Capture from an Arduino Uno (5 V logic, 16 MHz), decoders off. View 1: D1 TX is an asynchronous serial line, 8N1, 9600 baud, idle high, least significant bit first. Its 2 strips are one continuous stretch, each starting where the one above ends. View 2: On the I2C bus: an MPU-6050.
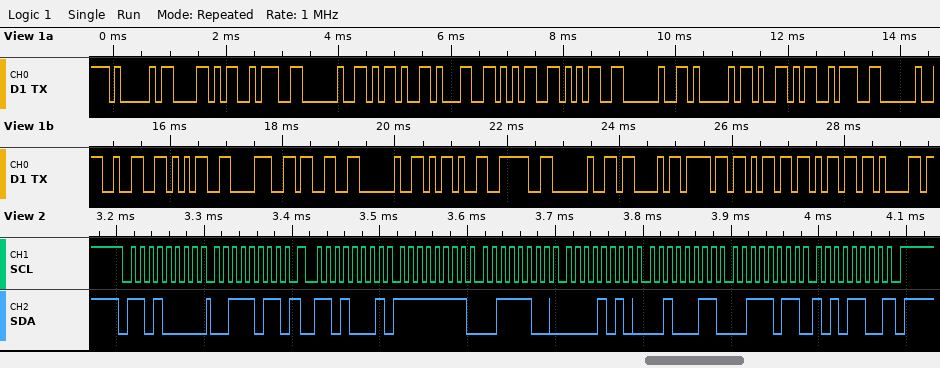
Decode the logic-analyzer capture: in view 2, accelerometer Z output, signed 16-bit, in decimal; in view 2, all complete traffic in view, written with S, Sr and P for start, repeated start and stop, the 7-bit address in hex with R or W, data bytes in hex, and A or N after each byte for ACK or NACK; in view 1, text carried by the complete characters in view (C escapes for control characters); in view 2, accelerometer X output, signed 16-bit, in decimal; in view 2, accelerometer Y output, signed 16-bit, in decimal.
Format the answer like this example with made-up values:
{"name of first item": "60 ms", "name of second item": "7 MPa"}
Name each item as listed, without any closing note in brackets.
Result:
{"in view 2, accelerometer Z output, signed 16-bit, in decimal": "15276", "in view 2, all complete traffic in view, written with S, Sr and P for start, repeated start and stop, the 7-bit address in hex with R or W, data bytes in hex, and A or N after each byte for ACK or NACK": "S 68W A 3B A Sr 68R A FF A 3C A 0A A 23 A 3B A AC N P", "in view 1, text carried by the complete characters in view": "\"AX: -155 AY: 2583 -> Comma\"", "in view 2, accelerometer X output, signed 16-bit, in decimal": "-196", "in view 2, accelerometer Y output, signed 16-bit, in decimal": "2595"}
